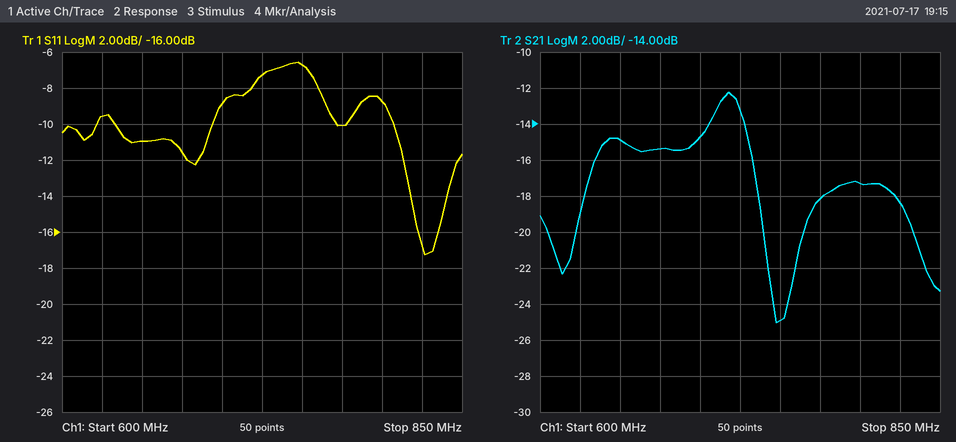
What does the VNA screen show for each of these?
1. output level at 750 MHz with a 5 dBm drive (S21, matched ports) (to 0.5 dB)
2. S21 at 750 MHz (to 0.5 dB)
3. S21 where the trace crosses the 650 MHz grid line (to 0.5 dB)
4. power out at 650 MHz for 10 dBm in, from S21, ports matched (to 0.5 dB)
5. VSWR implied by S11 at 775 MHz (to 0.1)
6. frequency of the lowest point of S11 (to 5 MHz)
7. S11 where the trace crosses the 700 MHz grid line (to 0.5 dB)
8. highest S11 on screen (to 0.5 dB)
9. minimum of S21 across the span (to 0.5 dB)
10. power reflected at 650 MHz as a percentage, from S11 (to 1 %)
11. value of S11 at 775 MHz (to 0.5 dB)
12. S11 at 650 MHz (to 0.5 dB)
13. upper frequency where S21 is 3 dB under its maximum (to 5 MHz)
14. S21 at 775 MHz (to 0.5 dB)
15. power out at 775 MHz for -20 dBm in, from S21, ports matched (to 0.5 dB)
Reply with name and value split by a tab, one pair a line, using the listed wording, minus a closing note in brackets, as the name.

output level at 750 MHz with a 5 dBm drive (S21, matched ports)	-20.0 dBm
S21 at 750 MHz	-25.0 dB
S21 where the trace crosses the 650 MHz grid line	-15.0 dB
power out at 650 MHz for 10 dBm in, from S21, ports matched	-5.0 dBm
VSWR implied by S11 at 775 MHz	1.9
frequency of the lowest point of S11	825 MHz
S11 where the trace crosses the 700 MHz grid line	-9.0 dB
highest S11 on screen	-6.5 dB
minimum of S21 across the span	-25.0 dB
power reflected at 650 MHz as a percentage, from S11	8 %
value of S11 at 775 MHz	-10.0 dB
S11 at 650 MHz	-11.0 dB
upper frequency where S21 is 3 dB under its maximum	730 MHz
S21 at 775 MHz	-18.0 dB
power out at 775 MHz for -20 dBm in, from S21, ports matched	-38.0 dBm
